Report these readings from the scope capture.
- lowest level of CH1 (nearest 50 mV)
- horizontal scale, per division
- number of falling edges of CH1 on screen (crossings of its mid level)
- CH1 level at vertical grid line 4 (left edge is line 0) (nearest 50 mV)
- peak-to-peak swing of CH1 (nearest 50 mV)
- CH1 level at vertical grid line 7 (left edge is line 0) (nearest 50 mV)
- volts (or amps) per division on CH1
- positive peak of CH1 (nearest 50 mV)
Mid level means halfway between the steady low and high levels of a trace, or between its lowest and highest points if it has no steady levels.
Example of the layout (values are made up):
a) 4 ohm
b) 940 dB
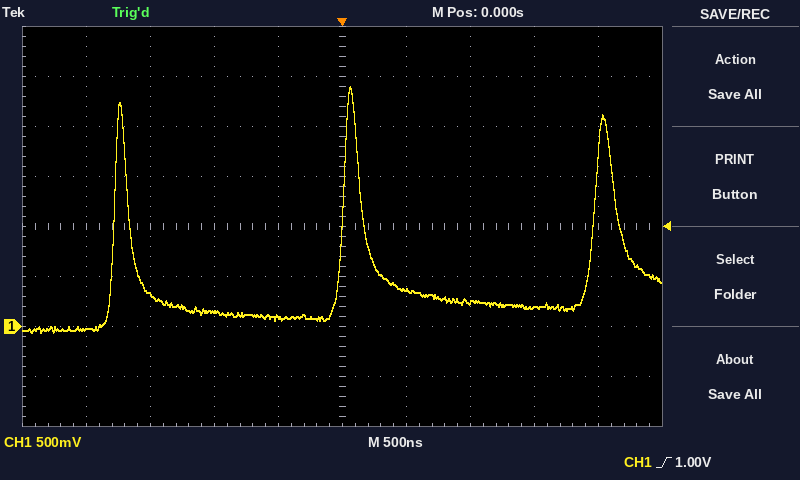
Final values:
a) -50 mV
b) 500 ns
c) 3
d) 100 mV
e) 2.45 V
f) 250 mV
g) 500 mV
h) 2.40 V
